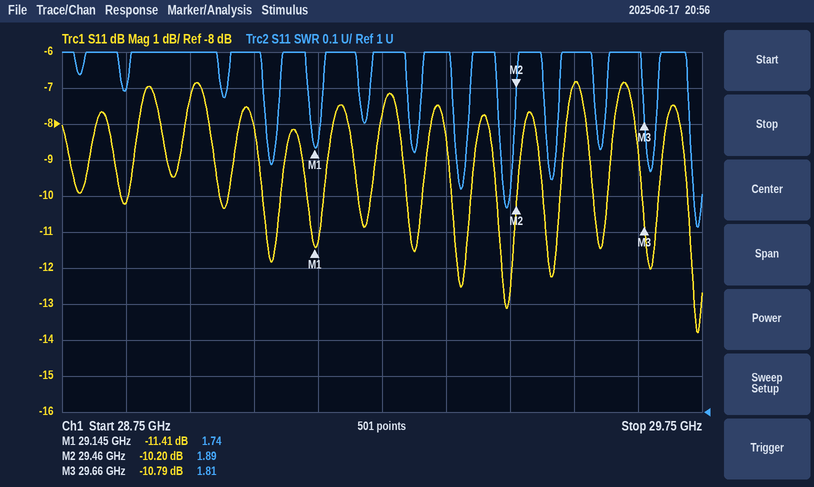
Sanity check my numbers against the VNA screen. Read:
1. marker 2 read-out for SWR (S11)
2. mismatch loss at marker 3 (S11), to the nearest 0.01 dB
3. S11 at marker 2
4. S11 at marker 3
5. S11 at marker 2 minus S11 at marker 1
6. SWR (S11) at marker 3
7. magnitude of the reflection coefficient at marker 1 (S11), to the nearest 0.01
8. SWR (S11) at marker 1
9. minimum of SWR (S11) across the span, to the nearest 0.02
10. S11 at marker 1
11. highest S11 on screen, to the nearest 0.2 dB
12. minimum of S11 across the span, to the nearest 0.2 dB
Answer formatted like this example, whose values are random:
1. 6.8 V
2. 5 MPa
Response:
1. 1.89
2. 0.38 dB
3. -10.20 dB
4. -10.79 dB
5. 1.21 dB
6. 1.81
7. 0.27
8. 1.74
9. 1.52
10. -11.41 dB
11. -6.8 dB
12. -13.8 dB
